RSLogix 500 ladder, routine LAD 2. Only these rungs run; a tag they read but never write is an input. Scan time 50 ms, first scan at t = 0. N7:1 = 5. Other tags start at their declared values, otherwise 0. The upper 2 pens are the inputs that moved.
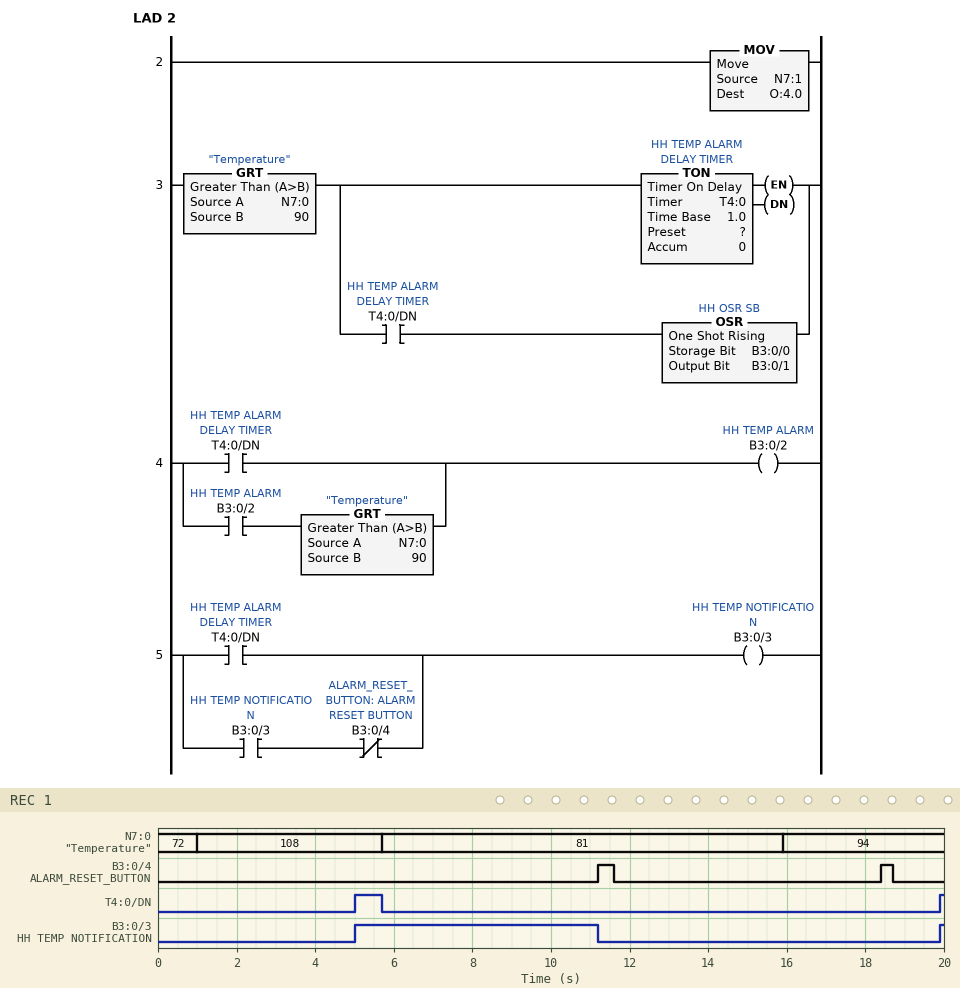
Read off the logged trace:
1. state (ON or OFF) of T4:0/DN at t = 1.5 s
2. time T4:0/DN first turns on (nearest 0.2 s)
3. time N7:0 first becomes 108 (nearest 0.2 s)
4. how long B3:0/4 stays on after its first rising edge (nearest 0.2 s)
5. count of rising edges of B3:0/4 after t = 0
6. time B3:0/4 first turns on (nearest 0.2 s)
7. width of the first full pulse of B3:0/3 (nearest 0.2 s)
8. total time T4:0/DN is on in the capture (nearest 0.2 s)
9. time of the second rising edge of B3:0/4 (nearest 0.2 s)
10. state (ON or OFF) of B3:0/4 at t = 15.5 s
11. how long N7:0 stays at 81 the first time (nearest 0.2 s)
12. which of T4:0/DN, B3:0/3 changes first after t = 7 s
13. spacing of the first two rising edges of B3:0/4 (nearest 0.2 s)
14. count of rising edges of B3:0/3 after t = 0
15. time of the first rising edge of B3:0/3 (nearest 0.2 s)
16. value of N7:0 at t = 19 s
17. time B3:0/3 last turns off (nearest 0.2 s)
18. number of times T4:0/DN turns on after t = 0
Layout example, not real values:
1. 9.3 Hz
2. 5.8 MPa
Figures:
1. OFF
2. 5.0 s
3. 1.0 s
4. 0.4 s
5. 2
6. 11.2 s
7. 6.2 s
8. 0.8 s
9. 18.4 s
10. OFF
11. 10.2 s
12. B3:0/3
13. 7.2 s
14. 2
15. 5.0 s
16. 94
17. 11.2 s
18. 2
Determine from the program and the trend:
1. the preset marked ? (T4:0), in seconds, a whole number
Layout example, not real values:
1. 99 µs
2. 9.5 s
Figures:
1. 4 s
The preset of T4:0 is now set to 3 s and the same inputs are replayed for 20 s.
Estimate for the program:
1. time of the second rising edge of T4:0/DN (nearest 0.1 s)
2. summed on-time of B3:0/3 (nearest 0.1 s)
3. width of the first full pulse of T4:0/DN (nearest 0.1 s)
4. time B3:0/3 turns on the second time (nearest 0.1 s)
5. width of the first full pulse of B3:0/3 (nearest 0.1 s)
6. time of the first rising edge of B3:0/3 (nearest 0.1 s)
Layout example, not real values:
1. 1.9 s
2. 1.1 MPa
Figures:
1. 18.9 s
2. 8.3 s
3. 1.7 s
4. 18.9 s
5. 7.2 s
6. 4.0 s
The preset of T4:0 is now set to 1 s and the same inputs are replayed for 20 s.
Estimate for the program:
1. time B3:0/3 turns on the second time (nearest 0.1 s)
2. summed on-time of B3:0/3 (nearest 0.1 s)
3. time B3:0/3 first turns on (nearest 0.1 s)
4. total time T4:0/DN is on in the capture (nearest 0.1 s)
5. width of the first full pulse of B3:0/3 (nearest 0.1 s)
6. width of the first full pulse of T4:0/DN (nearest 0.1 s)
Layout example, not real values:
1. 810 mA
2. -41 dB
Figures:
1. 16.9 s
2. 12.3 s
3. 2.0 s
4. 6.8 s
5. 9.2 s
6. 3.7 s
